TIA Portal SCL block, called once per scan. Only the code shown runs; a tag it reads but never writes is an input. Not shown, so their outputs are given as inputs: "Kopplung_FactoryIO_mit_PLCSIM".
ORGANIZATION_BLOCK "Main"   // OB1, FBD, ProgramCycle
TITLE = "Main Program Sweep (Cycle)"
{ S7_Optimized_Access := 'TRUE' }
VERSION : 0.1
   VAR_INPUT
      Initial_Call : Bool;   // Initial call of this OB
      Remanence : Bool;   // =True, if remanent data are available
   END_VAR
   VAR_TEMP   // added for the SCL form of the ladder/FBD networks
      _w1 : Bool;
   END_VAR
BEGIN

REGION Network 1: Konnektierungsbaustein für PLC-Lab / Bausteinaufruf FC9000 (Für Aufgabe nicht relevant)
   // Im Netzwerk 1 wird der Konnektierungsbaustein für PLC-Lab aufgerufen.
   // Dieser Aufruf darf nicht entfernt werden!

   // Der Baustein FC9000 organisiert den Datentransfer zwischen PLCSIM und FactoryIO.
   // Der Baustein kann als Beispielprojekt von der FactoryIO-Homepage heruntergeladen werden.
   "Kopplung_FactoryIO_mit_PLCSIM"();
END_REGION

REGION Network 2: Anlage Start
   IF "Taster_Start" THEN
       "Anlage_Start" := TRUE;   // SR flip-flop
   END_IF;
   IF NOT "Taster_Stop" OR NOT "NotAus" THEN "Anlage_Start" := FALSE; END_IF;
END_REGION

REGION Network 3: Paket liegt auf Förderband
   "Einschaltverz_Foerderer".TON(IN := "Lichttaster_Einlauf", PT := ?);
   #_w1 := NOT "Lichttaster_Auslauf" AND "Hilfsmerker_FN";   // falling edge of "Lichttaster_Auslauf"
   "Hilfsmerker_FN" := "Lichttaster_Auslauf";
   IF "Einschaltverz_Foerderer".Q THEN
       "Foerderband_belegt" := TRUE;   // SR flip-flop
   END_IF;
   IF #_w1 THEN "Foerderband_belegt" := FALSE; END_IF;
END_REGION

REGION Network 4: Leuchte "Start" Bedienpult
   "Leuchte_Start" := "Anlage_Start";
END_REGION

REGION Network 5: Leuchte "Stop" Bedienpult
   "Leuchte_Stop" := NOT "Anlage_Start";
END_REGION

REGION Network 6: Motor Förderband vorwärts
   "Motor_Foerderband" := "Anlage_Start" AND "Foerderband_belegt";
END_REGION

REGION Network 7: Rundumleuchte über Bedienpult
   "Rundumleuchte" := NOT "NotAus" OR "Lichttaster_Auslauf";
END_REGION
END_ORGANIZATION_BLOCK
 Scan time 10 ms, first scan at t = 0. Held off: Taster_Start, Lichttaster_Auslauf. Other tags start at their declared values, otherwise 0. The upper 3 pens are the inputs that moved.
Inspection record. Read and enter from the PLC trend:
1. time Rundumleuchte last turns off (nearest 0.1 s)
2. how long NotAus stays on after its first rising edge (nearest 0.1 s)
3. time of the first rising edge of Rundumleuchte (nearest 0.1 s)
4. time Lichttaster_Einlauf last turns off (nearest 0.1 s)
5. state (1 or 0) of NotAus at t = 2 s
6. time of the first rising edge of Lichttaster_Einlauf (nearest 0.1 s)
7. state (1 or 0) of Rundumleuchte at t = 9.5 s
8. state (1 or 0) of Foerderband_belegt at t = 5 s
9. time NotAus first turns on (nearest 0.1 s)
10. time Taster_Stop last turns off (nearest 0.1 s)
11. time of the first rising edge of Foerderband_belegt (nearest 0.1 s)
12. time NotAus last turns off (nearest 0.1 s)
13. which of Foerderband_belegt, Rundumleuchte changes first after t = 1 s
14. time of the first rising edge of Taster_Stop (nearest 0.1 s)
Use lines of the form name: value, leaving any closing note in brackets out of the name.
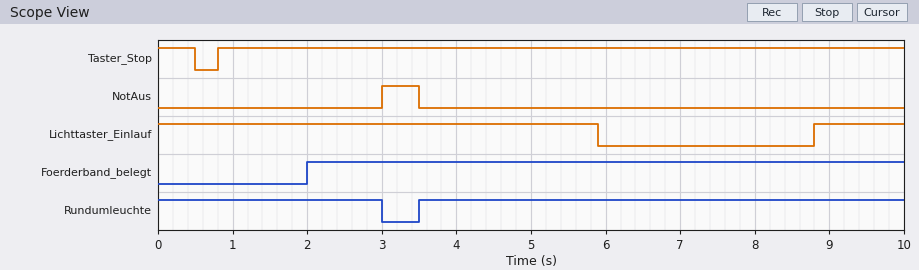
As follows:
time Rundumleuchte last turns off: 3.0 s
how long NotAus stays on after its first rising edge: 0.5 s
time of the first rising edge of Rundumleuchte: 3.5 s
time Lichttaster_Einlauf last turns off: 5.9 s
state (1 or 0) of NotAus at t = 2 s: 0
time of the first rising edge of Lichttaster_Einlauf: 8.8 s
state (1 or 0) of Rundumleuchte at t = 9.5 s: 1
state (1 or 0) of Foerderband_belegt at t = 5 s: 1
time NotAus first turns on: 3.0 s
time Taster_Stop last turns off: 0.5 s
time of the first rising edge of Foerderband_belegt: 2.0 s
time NotAus last turns off: 3.5 s
which of Foerderband_belegt, Rundumleuchte changes first after t = 1 s: Foerderband_belegt
time of the first rising edge of Taster_Stop: 0.8 s
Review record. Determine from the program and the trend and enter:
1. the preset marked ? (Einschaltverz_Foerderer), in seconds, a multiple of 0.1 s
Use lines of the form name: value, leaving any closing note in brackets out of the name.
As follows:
the preset marked ? (Einschaltverz_Foerderer), in seconds, a multiple of 0.1 s: 2.0 s
